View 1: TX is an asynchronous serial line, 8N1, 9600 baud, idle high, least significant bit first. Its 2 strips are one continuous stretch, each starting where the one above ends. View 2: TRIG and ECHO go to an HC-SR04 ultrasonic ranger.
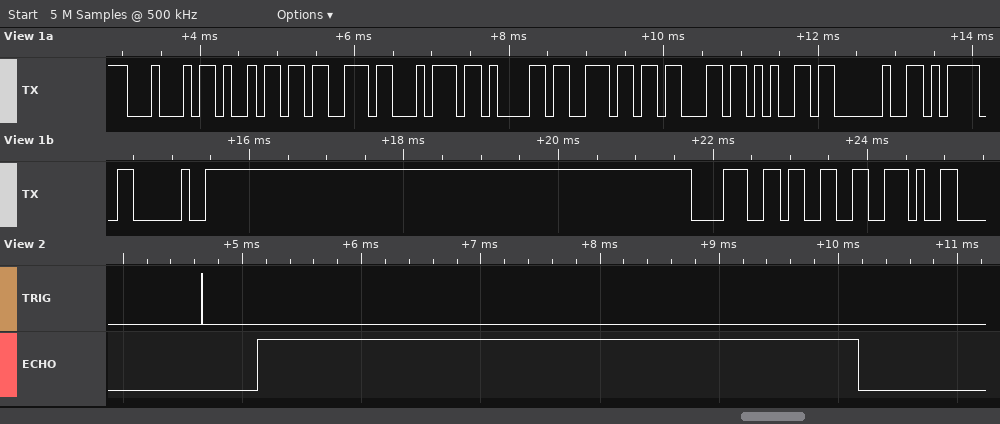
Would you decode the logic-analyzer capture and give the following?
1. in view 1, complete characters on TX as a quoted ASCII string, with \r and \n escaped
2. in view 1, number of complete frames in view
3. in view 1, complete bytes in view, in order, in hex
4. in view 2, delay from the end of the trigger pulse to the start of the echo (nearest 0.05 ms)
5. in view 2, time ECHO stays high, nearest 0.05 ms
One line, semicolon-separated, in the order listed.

"Distance = 83."; 14; 0x44 0x69 0x73 0x74 0x61 0x6E 0x63 0x65 0x20 0x3D 0x20 0x38 0x33 0x2E; 0.45 ms; 5.05 ms
